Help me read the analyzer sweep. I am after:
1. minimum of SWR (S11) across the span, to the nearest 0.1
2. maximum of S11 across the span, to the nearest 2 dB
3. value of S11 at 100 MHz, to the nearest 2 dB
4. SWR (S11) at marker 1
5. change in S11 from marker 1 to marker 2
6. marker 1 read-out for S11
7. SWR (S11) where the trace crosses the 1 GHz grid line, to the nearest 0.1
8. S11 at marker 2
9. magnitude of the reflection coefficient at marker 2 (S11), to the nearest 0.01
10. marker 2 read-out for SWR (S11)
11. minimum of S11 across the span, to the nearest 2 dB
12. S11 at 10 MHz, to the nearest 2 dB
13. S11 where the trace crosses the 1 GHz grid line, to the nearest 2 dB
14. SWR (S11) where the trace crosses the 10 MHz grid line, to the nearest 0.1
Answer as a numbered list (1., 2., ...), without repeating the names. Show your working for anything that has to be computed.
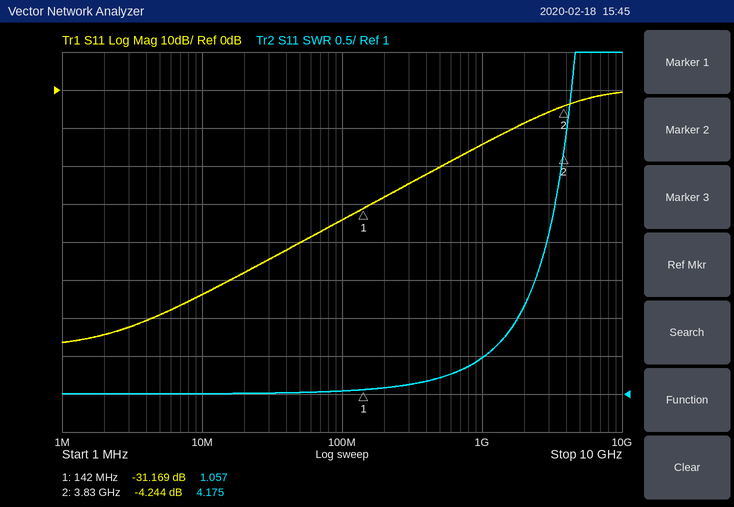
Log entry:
1. 1.0
2. 0 dB
3. -34 dB
4. 1.057
5. -4.244 − (-31.169) = 26.925 dB
6. -31.169 dB
7. 1.5
8. -4.244 dB
9. 10^(-4.244/20) ≈ 0.61
10. 4.175
11. -66 dB
12. -54 dB
13. -14 dB
14. 1.0
